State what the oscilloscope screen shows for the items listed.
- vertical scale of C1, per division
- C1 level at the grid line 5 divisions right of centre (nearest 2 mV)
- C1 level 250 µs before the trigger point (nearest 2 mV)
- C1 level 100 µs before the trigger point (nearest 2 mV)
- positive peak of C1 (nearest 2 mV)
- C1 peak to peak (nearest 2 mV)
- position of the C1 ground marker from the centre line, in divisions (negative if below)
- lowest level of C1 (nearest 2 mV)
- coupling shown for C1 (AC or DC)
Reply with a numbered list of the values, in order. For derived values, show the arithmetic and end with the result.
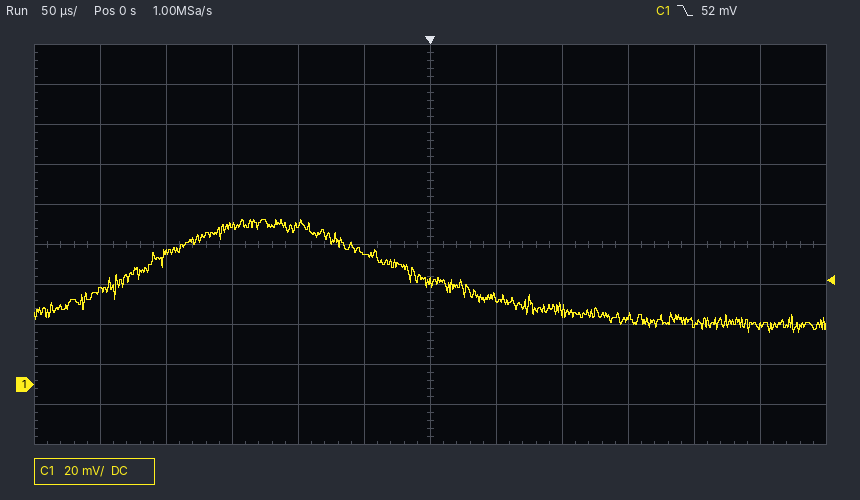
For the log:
1. 20 mV
2. 30 mV
3. 46 mV
4. 80 mV
5. 82 mV
6. 82 mV − (26 mV) = 56 mV
7. -3.5 div
8. 26 mV
9. DC
